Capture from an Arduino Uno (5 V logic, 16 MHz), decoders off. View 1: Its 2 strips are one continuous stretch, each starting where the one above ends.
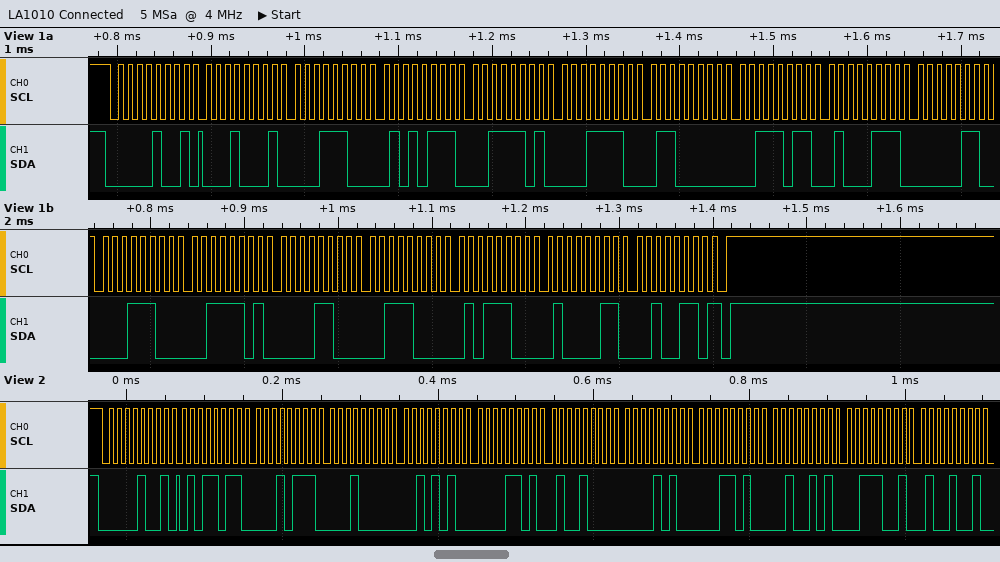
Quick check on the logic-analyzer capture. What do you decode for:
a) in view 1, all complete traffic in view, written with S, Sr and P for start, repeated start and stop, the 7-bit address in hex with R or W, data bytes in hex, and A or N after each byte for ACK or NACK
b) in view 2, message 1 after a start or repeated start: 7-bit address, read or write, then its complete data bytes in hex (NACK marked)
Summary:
S 04R A 11 A 1C A 57 A 3D A 1E A 60 A 3B A 47 A 06 A 1C A 3D A 0C A 38 A 5C A 43 A 26 N P
0x04 read: 5B 17 10 2A 0D 48 0A 1A 25 39 49
